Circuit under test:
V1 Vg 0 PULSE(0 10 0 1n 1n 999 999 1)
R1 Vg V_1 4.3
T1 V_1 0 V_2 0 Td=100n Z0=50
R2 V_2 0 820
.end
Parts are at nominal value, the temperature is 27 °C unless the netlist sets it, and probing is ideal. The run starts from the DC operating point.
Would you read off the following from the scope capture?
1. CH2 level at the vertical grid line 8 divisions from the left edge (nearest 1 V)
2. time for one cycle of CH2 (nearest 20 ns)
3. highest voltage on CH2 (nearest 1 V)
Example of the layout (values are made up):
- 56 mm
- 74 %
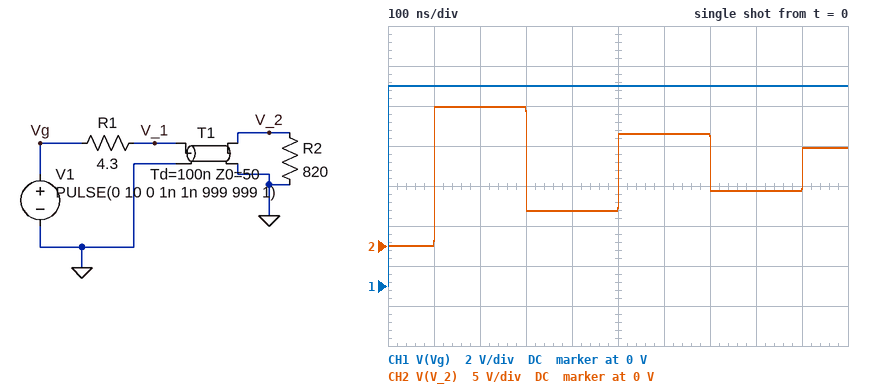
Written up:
- 7 V
- 400 ns
- 17 V
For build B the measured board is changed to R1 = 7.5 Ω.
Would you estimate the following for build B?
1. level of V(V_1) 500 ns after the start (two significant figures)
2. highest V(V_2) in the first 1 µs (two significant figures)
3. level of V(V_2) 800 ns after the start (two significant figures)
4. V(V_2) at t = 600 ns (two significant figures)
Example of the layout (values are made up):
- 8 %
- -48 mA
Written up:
- 9.4 V
- 16 V
- 8.1 V
- 13 V
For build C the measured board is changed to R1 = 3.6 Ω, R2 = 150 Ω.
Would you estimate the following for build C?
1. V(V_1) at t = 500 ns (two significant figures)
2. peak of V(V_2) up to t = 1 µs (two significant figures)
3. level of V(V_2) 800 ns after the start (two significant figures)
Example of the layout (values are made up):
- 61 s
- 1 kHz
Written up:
- 9.7 V
- 14 V
- 9.4 V
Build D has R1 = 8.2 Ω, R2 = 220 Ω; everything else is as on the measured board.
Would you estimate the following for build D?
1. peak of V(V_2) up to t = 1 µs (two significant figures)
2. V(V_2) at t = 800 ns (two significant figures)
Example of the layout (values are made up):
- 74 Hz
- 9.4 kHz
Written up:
- 14 V
- 9.2 V
